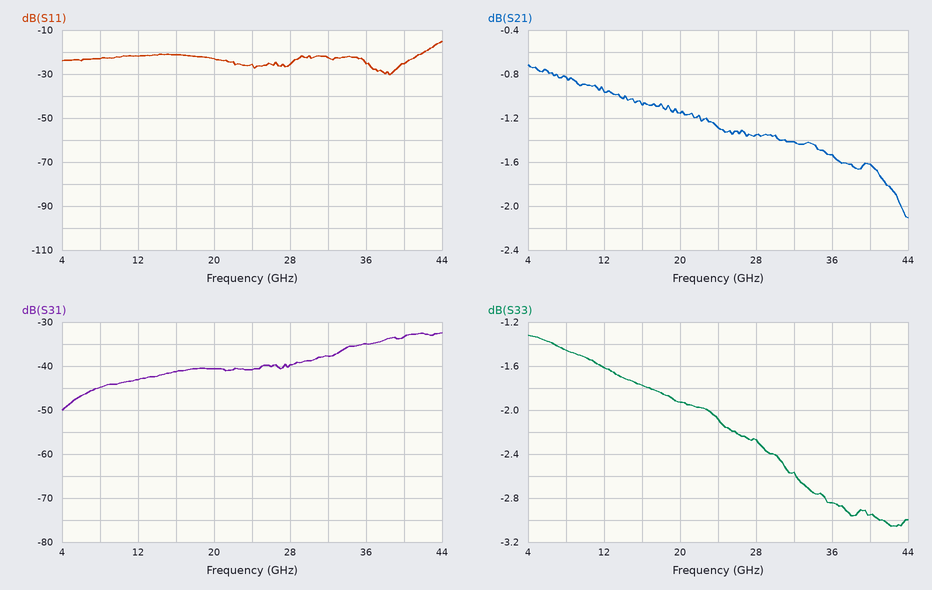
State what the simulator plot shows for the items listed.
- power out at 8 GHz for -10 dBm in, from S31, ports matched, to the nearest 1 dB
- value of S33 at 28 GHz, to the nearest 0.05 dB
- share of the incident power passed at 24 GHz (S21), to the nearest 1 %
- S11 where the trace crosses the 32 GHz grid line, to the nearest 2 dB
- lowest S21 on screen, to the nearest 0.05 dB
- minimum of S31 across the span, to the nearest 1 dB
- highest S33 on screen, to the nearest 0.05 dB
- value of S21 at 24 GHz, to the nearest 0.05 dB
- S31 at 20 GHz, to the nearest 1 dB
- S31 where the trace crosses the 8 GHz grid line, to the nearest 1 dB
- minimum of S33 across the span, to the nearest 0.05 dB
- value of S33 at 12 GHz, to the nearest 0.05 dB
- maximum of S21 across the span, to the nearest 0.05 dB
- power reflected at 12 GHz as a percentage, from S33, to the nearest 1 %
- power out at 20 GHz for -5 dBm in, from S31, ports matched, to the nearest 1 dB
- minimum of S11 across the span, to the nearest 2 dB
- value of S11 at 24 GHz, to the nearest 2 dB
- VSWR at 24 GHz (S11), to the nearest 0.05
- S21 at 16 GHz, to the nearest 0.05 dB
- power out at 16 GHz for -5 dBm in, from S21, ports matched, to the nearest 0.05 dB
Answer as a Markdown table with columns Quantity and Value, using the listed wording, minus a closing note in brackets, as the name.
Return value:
| Quantity | Value |
|---|---|
| power out at 8 GHz for -10 dBm in, from S31, ports matched, to the nearest 1 dB | -55 dBm |
| value of S33 at 28 GHz, to the nearest 0.05 dB | -2.25 dB |
| share of the incident power passed at 24 GHz (S21), to the nearest 1 % | 74 % |
| S11 where the trace crosses the 32 GHz grid line, to the nearest 2 dB | -22 dB |
| lowest S21 on screen, to the nearest 0.05 dB | -2.10 dB |
| minimum of S31 across the span, to the nearest 1 dB | -50 dB |
| highest S33 on screen, to the nearest 0.05 dB | -1.30 dB |
| value of S21 at 24 GHz, to the nearest 0.05 dB | -1.30 dB |
| S31 at 20 GHz, to the nearest 1 dB | -41 dB |
| S31 where the trace crosses the 8 GHz grid line, to the nearest 1 dB | -45 dB |
| minimum of S33 across the span, to the nearest 0.05 dB | -3.05 dB |
| value of S33 at 12 GHz, to the nearest 0.05 dB | -1.60 dB |
| maximum of S21 across the span, to the nearest 0.05 dB | -0.70 dB |
| power reflected at 12 GHz as a percentage, from S33, to the nearest 1 % | 69 % |
| power out at 20 GHz for -5 dBm in, from S31, ports matched, to the nearest 1 dB | -46 dBm |
| minimum of S11 across the span, to the nearest 2 dB | -30 dB |
| value of S11 at 24 GHz, to the nearest 2 dB | -26 dB |
| VSWR at 24 GHz (S11), to the nearest 0.05 | 1.10 |
| S21 at 16 GHz, to the nearest 0.05 dB | -1.10 dB |
| power out at 16 GHz for -5 dBm in, from S21, ports matched, to the nearest 0.05 dB | -6.10 dBm |
